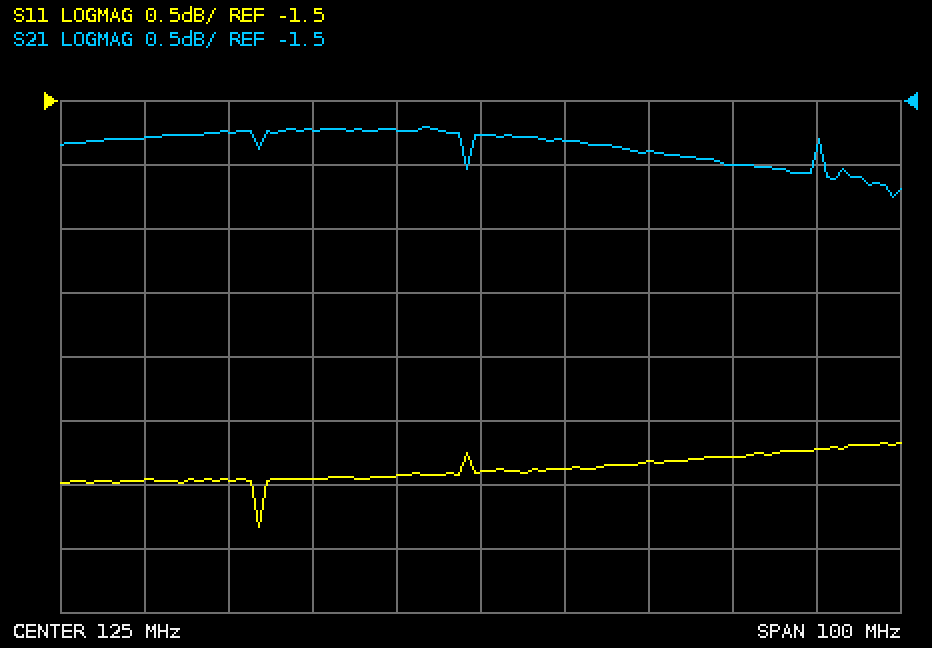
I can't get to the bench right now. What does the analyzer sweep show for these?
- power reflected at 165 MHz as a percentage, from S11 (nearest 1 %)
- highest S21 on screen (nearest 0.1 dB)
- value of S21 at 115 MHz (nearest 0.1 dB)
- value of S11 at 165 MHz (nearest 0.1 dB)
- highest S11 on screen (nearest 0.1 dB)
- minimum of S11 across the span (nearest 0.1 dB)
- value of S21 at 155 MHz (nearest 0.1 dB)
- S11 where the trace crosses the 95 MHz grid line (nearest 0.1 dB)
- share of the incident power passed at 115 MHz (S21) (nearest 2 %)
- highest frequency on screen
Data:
38 %
-1.7 dB
-1.7 dB
-4.2 dB
-4.2 dB
-4.8 dB
-2.0 dB
-4.5 dB
68 %
175 MHz
